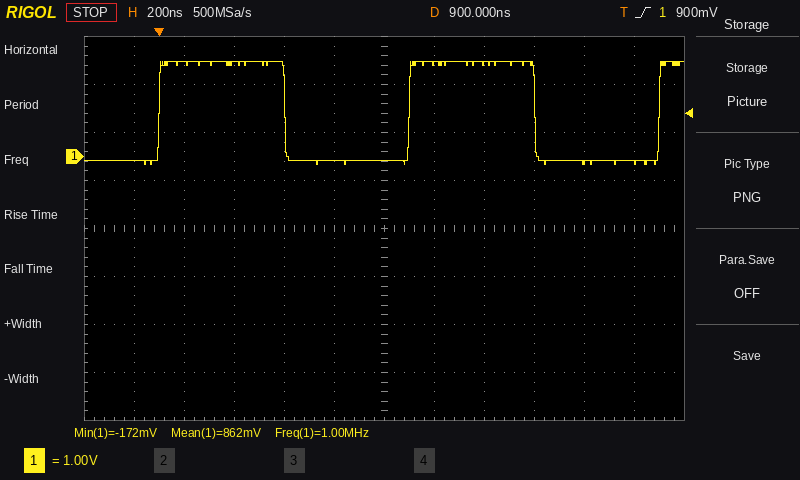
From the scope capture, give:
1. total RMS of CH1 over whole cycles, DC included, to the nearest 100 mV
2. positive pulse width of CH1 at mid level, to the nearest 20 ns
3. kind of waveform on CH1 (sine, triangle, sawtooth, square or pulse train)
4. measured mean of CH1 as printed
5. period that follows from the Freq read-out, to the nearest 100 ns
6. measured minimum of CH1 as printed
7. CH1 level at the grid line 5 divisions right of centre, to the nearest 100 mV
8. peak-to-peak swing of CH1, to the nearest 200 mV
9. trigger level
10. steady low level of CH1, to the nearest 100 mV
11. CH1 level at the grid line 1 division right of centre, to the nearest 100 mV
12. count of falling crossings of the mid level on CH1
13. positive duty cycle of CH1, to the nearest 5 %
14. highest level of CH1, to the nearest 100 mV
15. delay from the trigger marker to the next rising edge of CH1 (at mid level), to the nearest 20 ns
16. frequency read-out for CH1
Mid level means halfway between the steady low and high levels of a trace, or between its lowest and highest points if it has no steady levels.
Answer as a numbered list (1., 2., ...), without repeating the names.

1. 1.4 V
2. 500 ns
3. square
4. 862 mV
5. 1.0 µs
6. -172 mV
7. -100 mV
8. 2.2 V
9. 900 mV
10. -100 mV
11. 1.9 V
12. 2
13. 50 %
14. 2.0 V
15. 1.00 µs
16. 1.00 MHz
